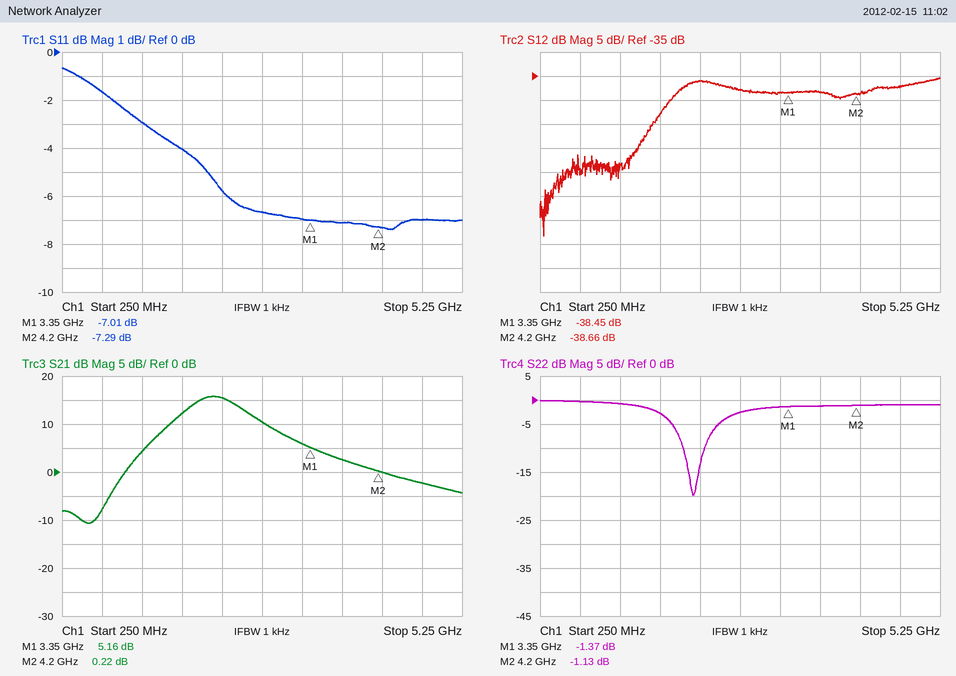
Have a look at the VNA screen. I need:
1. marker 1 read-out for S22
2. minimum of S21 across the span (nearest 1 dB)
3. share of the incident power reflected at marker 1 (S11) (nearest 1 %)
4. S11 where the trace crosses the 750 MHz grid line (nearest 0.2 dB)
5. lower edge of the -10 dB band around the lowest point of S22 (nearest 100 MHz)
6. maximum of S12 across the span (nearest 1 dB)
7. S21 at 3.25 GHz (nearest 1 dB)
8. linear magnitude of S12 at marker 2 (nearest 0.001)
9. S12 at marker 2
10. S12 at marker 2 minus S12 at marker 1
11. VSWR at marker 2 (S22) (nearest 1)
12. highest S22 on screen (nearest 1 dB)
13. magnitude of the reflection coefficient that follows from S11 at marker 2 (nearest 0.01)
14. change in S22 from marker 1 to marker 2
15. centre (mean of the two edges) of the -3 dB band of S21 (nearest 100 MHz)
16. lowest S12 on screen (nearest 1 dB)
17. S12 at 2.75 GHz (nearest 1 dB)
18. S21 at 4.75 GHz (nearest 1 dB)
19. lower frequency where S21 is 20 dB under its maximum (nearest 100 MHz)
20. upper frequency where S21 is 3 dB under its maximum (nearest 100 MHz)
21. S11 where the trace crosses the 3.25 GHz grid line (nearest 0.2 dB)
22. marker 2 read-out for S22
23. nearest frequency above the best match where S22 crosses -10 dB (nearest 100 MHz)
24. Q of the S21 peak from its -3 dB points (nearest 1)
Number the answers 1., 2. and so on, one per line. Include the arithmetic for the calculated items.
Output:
1. -1.37 dB
2. -11 dB
3. 10^(-7.01/10) ≈ 20 %
4. -1.6 dB
5. 2.0 GHz
6. -35 dB
7. 6 dB
8. 10^(-38.66/20) ≈ 0.012
9. -38.66 dB
10. -38.66 − (-38.45) = -0.21 dB
11. (1 + 0.8780)/(1 − 0.8780) ≈ 15
12. 0 dB
13. 10^(-7.29/20) ≈ 0.43
14. -1.13 − (-1.37) = 0.24 dB
15. 2.2 GHz
16. -68 dB
17. -38 dB
18. -2 dB
19. 900 MHz
20. 2.5 GHz
21. -7.0 dB
22. -1.13 dB
23. 2.3 GHz
24. 2.15 GHz / 700 MHz ≈ 3
